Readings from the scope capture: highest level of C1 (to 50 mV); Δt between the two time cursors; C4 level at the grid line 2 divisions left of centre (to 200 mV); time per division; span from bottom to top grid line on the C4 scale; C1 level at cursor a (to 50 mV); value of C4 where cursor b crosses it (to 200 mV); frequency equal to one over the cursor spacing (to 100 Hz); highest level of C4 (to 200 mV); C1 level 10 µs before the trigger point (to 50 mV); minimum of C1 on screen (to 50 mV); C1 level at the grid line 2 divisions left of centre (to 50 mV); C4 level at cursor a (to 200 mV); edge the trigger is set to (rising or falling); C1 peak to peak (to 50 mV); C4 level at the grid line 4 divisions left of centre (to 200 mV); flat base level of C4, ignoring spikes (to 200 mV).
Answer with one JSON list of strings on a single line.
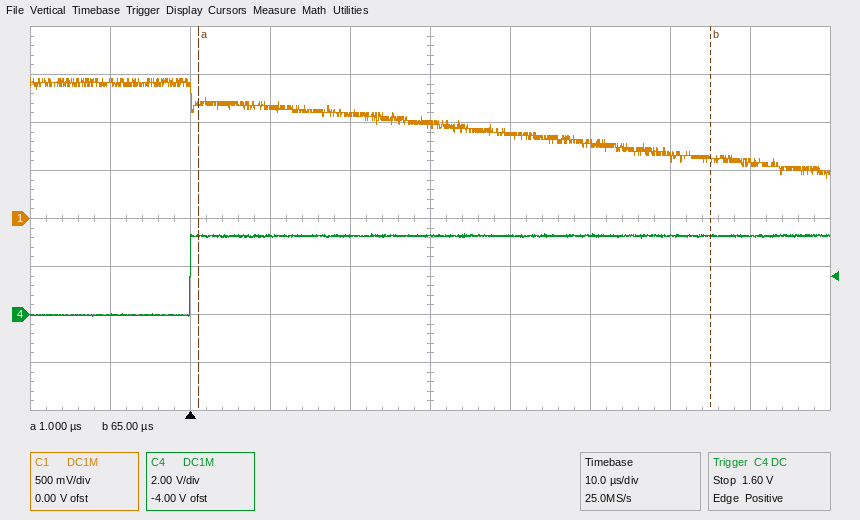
["1.45 V", "64 µs", "3.2 V", "10 µs", "16 V", "1.20 V", "3.2 V", "15.6 kHz", "3.4 V", "1.40 V", "400 mV", "1.15 V", "3.2 V", "rising", "1.05 V", "0.0 V", "0.0 V"]
